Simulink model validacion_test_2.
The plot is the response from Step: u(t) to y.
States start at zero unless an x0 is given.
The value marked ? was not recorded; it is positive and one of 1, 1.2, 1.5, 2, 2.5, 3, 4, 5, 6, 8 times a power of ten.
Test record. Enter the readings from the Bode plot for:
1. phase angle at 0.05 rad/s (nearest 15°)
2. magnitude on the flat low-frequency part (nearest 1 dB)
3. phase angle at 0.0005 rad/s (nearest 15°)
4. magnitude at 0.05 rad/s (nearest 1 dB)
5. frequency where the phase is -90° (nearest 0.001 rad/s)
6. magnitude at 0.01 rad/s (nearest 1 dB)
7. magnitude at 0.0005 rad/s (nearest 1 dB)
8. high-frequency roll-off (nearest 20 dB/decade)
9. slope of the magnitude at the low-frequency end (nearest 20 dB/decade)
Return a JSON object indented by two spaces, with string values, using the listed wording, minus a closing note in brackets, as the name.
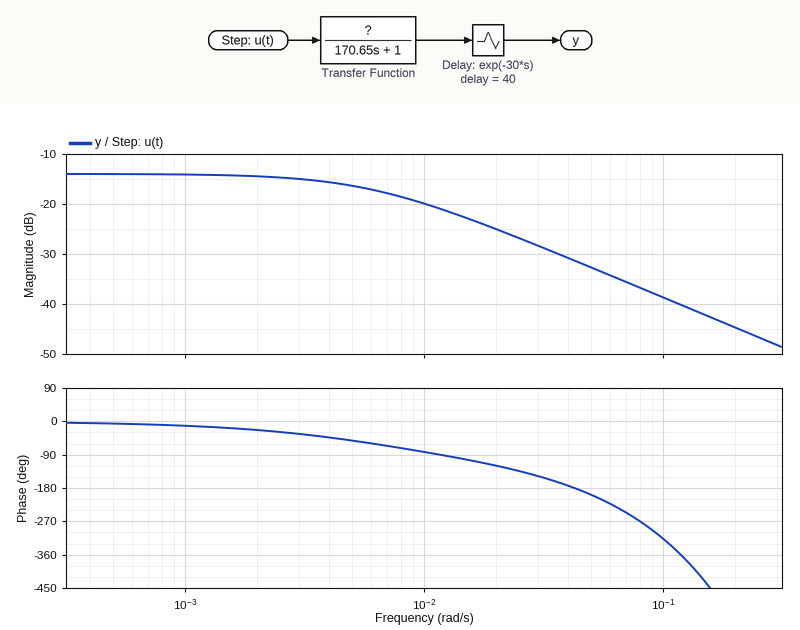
{
  "phase angle at 0.05 rad/s": "-195°",
  "magnitude on the flat low-frequency part": "-14 dB",
  "phase angle at 0.0005 rad/s": "0°",
  "magnitude at 0.05 rad/s": "-33 dB",
  "frequency where the phase is -90°": "0.012 rad/s",
  "magnitude at 0.01 rad/s": "-20 dB",
  "magnitude at 0.0005 rad/s": "-14 dB",
  "high-frequency roll-off": "-20 dB/decade",
  "slope of the magnitude at the low-frequency end": "0 dB/decade"
}
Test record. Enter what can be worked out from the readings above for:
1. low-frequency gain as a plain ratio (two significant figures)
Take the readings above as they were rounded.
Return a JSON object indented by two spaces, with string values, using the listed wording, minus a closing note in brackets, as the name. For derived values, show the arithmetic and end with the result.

{
  "low-frequency gain as a plain ratio": "10^(-14 / 20) = 0.20"
}
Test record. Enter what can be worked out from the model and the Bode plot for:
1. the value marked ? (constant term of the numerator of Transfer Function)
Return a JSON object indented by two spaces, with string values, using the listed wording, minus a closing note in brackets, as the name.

{
  "the value marked ?": "0.2"
}
